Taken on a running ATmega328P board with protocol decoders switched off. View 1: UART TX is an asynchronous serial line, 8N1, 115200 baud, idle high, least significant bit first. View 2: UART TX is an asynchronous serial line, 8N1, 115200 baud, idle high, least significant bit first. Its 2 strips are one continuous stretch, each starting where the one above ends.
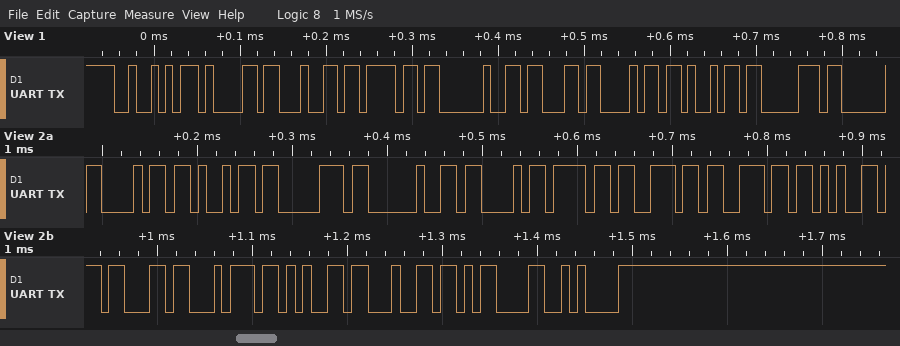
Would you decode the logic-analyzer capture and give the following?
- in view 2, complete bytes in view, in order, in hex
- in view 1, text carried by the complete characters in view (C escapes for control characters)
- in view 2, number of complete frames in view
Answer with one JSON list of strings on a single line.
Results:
["68 69 70 20 43 6F 6E 6E 65 63 74 65 64 0D 0A", "\"Rado chip\"", "15"]
